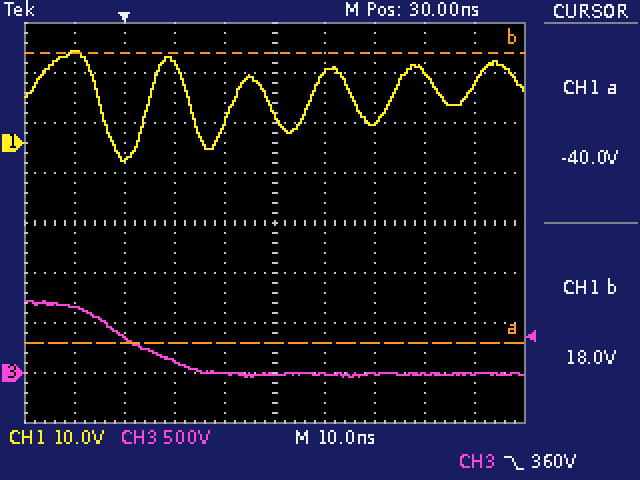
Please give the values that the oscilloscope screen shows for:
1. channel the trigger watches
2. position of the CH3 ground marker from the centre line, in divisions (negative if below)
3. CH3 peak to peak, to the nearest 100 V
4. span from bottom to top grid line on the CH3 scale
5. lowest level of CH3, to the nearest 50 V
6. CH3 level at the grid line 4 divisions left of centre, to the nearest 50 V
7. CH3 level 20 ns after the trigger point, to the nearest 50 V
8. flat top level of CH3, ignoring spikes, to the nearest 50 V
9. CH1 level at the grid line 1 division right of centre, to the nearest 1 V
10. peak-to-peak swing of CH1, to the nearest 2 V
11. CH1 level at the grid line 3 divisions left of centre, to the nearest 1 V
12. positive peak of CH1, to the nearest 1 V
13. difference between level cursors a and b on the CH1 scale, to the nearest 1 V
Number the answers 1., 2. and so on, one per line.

1. CH3
2. -3.0 div
3. 800 V
4. 4 kV
5. -50 V
6. 650 V
7. 0 V
8. 700 V
9. 14 V
10. 22 V
11. -3 V
12. 18 V
13. 58 V
